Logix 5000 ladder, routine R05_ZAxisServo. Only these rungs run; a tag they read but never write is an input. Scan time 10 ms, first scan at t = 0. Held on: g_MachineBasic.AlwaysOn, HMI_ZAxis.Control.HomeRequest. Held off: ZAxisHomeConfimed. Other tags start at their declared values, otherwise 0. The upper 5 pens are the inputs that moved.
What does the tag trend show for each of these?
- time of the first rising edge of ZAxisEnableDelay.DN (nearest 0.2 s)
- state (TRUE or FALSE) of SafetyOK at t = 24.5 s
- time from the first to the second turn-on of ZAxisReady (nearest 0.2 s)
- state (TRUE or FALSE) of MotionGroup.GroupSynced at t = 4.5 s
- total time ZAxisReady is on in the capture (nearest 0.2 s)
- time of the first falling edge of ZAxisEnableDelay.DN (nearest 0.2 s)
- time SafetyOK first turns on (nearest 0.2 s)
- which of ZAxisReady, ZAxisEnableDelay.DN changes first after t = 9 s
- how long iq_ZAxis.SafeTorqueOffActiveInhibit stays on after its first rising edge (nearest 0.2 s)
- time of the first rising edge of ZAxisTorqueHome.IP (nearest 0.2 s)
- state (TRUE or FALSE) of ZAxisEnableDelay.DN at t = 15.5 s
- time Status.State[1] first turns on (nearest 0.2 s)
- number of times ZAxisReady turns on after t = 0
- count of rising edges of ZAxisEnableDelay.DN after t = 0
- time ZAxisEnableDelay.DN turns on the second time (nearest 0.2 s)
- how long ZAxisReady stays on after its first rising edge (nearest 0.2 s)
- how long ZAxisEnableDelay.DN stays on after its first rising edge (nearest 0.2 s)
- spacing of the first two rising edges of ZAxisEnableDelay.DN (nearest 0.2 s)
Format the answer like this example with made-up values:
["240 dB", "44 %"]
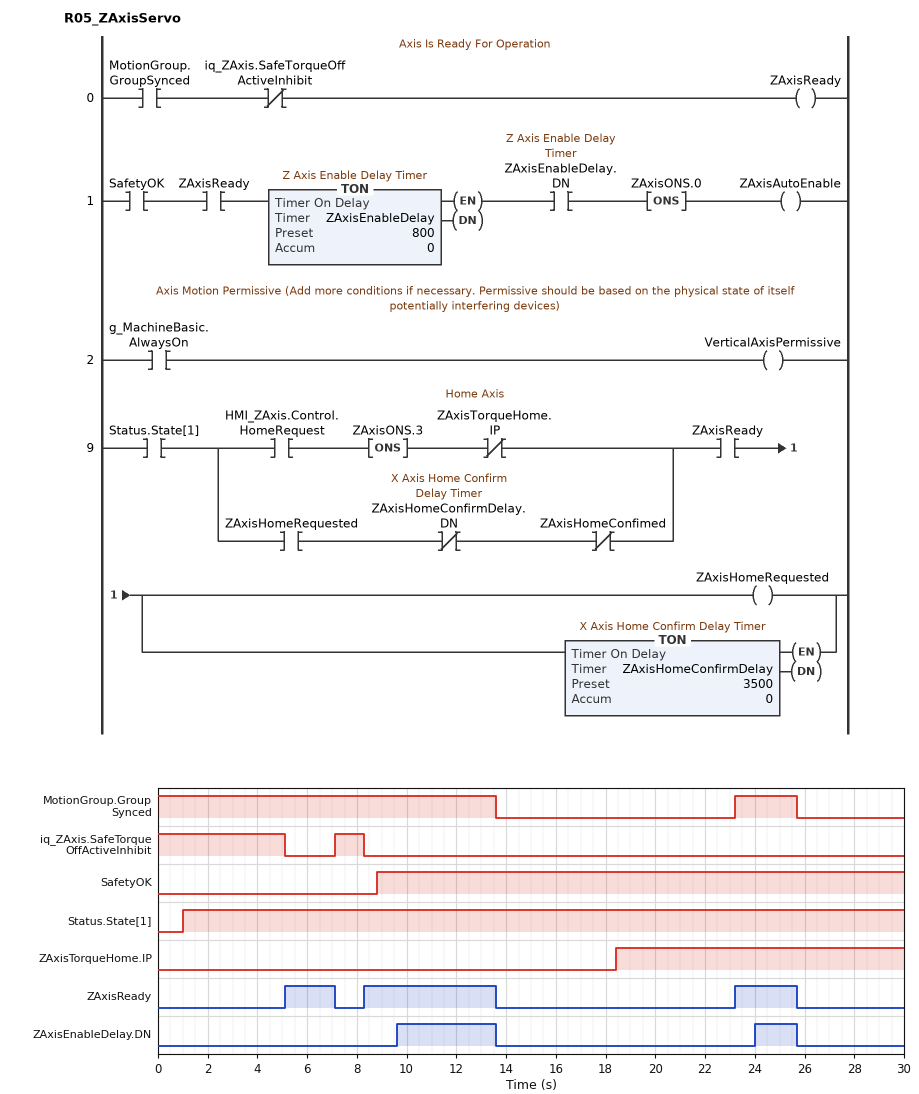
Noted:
["9.6 s", "TRUE", "3.2 s", "TRUE", "9.8 s", "13.6 s", "8.8 s", "ZAxisEnableDelay.DN", "1.2 s", "18.4 s", "FALSE", "1.0 s", "3", "2", "24.0 s", "2.0 s", "4.0 s", "14.4 s"]
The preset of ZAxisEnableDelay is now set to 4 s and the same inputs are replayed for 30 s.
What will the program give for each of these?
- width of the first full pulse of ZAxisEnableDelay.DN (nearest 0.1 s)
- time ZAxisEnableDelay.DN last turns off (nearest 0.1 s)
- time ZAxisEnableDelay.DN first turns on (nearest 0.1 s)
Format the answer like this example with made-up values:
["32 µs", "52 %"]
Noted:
["0.8 s", "13.6 s", "12.8 s"]
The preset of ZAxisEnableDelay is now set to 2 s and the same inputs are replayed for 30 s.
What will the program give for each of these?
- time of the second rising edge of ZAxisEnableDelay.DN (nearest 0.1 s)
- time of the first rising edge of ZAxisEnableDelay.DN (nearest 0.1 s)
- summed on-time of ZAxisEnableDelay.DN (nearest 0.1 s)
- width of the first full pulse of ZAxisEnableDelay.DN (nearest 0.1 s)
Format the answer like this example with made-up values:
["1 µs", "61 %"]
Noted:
["25.2 s", "10.8 s", "3.3 s", "2.8 s"]
